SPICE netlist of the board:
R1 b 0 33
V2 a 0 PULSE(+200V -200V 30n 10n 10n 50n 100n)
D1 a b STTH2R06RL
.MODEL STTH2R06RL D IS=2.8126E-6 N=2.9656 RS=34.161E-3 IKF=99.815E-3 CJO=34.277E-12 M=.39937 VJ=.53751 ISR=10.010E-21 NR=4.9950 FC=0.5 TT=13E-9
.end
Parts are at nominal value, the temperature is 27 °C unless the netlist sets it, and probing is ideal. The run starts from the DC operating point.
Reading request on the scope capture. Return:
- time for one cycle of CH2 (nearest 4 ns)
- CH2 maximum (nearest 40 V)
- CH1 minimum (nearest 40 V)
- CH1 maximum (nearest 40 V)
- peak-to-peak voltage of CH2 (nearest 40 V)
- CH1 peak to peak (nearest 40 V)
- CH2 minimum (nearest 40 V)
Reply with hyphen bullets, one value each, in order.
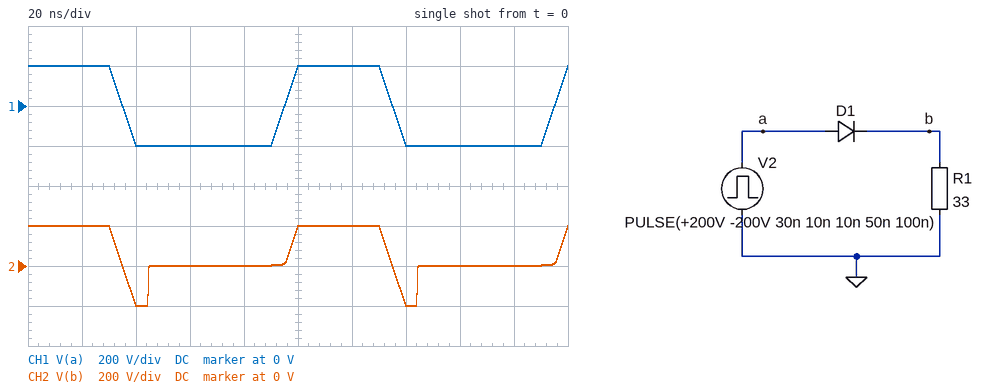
- 100 ns
- 200 V
- -200 V
- 200 V
- 400 V
- 400 V
- -200 V
